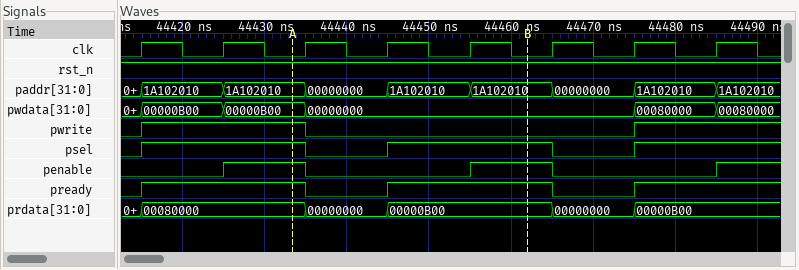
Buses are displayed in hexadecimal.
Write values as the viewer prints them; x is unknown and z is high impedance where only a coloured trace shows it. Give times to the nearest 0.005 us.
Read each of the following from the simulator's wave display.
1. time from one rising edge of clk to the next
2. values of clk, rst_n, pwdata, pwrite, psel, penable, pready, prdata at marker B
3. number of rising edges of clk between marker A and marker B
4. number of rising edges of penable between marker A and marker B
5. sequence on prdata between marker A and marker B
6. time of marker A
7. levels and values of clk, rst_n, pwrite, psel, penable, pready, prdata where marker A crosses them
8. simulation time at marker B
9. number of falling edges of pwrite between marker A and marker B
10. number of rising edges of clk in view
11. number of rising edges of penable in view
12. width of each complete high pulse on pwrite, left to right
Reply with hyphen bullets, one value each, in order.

- 0.01 us
- clk=0, rst_n=1, pwdata=00000000, pwrite=0, psel=1, penable=1, pready=1, prdata=00000B00
- 3
- 1
- 00080000, 00000000, 00000B00
- 44.435 us
- clk=0, rst_n=1, pwrite=1, psel=1, penable=1, pready=1, prdata=00080000
- 44.46 us
- 1
- 8
- 3
- 0.02 us
